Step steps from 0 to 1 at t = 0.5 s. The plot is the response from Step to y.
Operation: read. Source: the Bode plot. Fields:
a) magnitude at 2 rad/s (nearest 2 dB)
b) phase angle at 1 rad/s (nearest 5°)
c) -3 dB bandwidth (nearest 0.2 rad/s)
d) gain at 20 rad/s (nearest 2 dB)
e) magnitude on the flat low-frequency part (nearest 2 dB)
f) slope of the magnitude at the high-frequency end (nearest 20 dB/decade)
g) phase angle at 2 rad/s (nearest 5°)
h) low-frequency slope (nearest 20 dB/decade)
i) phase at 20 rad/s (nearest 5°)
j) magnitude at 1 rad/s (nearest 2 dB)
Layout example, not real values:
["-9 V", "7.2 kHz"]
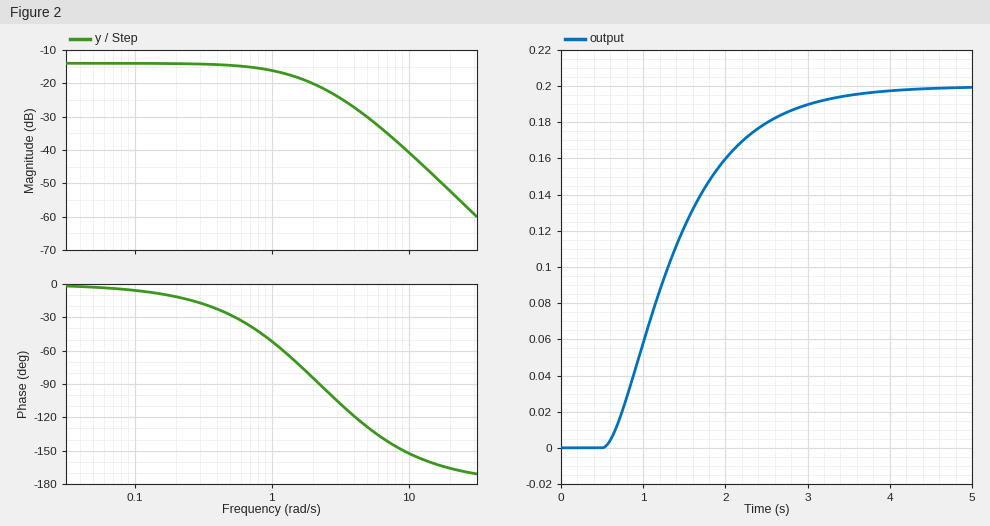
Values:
["-20 dB", "-50°", "1.2 rad/s", "-52 dB", "-14 dB", "-40 dB/decade", "-85°", "0 dB/decade", "-165°", "-16 dB"]
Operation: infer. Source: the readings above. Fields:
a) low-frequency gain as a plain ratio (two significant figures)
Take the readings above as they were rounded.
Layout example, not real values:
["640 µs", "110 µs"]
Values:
["0.20"]
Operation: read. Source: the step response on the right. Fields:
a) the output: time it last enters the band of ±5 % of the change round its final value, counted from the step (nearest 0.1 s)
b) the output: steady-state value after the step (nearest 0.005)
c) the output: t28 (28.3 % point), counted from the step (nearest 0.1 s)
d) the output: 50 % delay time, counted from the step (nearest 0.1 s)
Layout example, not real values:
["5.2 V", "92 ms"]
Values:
["2.5 s", "0.200", "0.5 s", "0.8 s"]
